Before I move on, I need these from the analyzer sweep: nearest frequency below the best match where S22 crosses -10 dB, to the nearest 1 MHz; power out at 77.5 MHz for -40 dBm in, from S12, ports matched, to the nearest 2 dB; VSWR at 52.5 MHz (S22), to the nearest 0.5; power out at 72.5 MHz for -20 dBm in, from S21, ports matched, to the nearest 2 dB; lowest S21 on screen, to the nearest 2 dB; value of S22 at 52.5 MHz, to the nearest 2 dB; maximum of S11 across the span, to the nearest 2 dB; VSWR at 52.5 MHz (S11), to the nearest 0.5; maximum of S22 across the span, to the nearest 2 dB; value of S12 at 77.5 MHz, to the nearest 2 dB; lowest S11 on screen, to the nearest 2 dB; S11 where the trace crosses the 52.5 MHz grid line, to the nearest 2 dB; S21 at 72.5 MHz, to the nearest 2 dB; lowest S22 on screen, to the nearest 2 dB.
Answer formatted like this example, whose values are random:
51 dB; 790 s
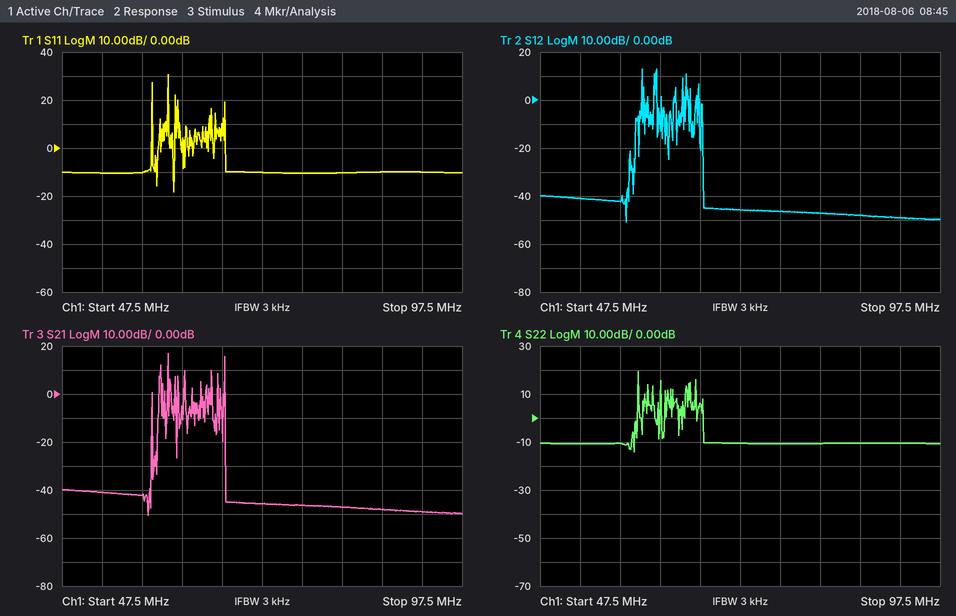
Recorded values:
59 MHz; -86 dBm; 2.0; -66 dBm; -50 dB; -10 dB; 30 dB; 2.0; 20 dB; -46 dB; -18 dB; -10 dB; -46 dB; -14 dB
